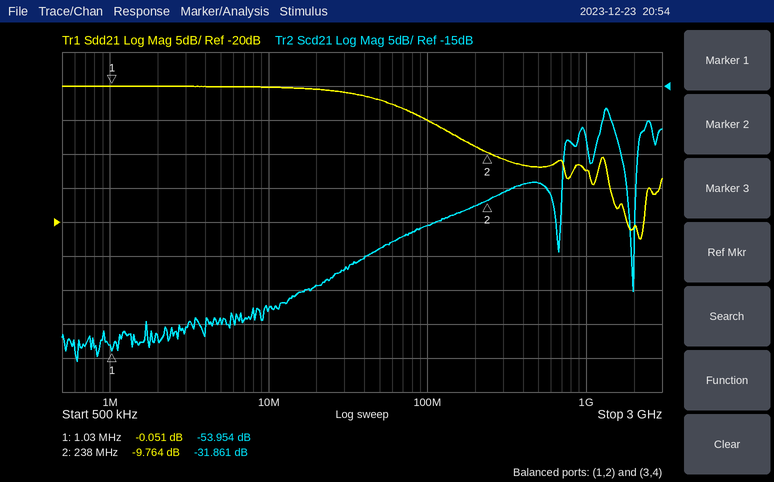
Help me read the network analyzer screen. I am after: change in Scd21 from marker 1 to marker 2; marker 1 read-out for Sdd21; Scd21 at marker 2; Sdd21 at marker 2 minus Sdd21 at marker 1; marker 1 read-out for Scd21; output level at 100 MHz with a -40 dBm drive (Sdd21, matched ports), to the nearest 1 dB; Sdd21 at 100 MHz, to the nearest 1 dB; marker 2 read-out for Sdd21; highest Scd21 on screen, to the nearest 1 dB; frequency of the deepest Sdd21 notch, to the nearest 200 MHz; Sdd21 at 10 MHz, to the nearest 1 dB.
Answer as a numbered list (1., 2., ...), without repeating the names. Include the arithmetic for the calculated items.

1. -31.861 − (-53.954) = 22.093 dB
2. -0.051 dB
3. -31.861 dB
4. -9.764 − (-0.051) = -9.713 dB
5. -53.954 dB
6. -40 dBm + (-5 dB) = -45 dBm
7. -5 dB
8. -9.764 dB
9. -18 dB
10. 2.2 GHz
11. 0 dB
